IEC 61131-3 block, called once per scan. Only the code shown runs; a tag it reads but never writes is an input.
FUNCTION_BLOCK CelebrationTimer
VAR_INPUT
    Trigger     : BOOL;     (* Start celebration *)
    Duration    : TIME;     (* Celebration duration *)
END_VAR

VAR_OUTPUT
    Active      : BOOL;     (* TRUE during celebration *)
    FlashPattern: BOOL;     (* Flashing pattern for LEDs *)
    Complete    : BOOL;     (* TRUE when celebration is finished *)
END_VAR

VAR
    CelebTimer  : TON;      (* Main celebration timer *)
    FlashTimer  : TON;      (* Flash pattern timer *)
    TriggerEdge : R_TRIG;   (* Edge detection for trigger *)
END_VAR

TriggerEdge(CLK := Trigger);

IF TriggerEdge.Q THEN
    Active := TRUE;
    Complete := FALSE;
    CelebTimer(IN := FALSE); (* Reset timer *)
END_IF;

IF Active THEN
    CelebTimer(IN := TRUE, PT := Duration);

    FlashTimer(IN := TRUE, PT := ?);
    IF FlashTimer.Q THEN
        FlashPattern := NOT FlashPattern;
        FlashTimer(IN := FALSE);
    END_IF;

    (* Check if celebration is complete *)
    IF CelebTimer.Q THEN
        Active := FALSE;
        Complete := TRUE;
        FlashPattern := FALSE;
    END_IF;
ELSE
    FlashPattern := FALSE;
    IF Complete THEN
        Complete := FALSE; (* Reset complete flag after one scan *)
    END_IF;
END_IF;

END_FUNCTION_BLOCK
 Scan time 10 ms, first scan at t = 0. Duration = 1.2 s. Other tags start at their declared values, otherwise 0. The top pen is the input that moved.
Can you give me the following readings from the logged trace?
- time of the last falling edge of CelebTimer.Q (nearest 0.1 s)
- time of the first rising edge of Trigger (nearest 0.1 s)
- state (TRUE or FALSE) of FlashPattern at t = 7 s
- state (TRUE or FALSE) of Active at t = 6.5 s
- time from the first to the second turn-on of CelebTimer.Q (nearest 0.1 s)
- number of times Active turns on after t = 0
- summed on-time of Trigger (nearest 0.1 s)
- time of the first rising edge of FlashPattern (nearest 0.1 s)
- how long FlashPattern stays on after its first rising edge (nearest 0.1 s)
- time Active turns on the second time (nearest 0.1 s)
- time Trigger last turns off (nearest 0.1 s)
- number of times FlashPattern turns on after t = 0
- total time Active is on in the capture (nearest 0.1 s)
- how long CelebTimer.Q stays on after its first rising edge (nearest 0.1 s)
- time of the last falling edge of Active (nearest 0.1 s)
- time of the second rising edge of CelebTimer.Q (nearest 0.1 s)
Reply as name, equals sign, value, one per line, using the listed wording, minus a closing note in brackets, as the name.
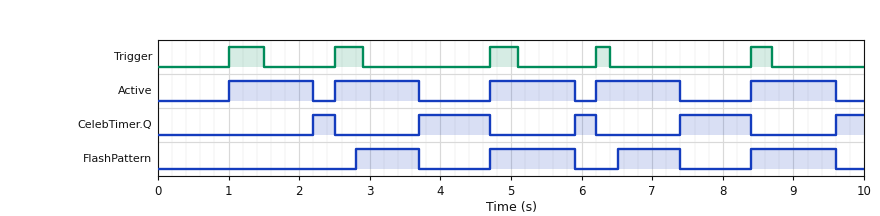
time of the last falling edge of CelebTimer.Q = 8.4 s
time of the first rising edge of Trigger = 1.0 s
state (TRUE or FALSE) of FlashPattern at t = 7 s = TRUE
state (TRUE or FALSE) of Active at t = 6.5 s = TRUE
time from the first to the second turn-on of CelebTimer.Q = 1.5 s
number of times Active turns on after t = 0 = 5
summed on-time of Trigger = 1.8 s
time of the first rising edge of FlashPattern = 2.8 s
how long FlashPattern stays on after its first rising edge = 0.9 s
time Active turns on the second time = 2.5 s
time Trigger last turns off = 8.7 s
number of times FlashPattern turns on after t = 0 = 4
total time Active is on in the capture = 6.0 s
how long CelebTimer.Q stays on after its first rising edge = 0.3 s
time of the last falling edge of Active = 9.6 s
time of the second rising edge of CelebTimer.Q = 3.7 s
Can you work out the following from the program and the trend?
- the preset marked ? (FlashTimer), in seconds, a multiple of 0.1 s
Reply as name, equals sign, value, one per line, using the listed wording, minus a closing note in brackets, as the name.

the preset marked ? (FlashTimer), in seconds, a multiple of 0.1 s = 1.8 s
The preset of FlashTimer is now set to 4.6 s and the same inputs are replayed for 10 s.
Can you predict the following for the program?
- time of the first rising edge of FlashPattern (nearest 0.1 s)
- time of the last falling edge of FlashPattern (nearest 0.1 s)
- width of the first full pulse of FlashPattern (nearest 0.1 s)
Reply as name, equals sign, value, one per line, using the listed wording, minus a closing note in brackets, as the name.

time of the first rising edge of FlashPattern = 5.6 s
time of the last falling edge of FlashPattern = 5.9 s
width of the first full pulse of FlashPattern = 0.3 s
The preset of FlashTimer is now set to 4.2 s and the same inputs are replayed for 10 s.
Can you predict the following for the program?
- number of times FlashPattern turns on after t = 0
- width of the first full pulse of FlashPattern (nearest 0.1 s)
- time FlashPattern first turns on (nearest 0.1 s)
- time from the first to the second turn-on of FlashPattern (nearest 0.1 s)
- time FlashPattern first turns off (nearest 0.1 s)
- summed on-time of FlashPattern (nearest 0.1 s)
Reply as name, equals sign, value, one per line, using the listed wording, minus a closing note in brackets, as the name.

number of times FlashPattern turns on after t = 0 = 2
width of the first full pulse of FlashPattern = 0.7 s
time FlashPattern first turns on = 5.2 s
time from the first to the second turn-on of FlashPattern = 4.2 s
time FlashPattern first turns off = 5.9 s
summed on-time of FlashPattern = 0.9 s
